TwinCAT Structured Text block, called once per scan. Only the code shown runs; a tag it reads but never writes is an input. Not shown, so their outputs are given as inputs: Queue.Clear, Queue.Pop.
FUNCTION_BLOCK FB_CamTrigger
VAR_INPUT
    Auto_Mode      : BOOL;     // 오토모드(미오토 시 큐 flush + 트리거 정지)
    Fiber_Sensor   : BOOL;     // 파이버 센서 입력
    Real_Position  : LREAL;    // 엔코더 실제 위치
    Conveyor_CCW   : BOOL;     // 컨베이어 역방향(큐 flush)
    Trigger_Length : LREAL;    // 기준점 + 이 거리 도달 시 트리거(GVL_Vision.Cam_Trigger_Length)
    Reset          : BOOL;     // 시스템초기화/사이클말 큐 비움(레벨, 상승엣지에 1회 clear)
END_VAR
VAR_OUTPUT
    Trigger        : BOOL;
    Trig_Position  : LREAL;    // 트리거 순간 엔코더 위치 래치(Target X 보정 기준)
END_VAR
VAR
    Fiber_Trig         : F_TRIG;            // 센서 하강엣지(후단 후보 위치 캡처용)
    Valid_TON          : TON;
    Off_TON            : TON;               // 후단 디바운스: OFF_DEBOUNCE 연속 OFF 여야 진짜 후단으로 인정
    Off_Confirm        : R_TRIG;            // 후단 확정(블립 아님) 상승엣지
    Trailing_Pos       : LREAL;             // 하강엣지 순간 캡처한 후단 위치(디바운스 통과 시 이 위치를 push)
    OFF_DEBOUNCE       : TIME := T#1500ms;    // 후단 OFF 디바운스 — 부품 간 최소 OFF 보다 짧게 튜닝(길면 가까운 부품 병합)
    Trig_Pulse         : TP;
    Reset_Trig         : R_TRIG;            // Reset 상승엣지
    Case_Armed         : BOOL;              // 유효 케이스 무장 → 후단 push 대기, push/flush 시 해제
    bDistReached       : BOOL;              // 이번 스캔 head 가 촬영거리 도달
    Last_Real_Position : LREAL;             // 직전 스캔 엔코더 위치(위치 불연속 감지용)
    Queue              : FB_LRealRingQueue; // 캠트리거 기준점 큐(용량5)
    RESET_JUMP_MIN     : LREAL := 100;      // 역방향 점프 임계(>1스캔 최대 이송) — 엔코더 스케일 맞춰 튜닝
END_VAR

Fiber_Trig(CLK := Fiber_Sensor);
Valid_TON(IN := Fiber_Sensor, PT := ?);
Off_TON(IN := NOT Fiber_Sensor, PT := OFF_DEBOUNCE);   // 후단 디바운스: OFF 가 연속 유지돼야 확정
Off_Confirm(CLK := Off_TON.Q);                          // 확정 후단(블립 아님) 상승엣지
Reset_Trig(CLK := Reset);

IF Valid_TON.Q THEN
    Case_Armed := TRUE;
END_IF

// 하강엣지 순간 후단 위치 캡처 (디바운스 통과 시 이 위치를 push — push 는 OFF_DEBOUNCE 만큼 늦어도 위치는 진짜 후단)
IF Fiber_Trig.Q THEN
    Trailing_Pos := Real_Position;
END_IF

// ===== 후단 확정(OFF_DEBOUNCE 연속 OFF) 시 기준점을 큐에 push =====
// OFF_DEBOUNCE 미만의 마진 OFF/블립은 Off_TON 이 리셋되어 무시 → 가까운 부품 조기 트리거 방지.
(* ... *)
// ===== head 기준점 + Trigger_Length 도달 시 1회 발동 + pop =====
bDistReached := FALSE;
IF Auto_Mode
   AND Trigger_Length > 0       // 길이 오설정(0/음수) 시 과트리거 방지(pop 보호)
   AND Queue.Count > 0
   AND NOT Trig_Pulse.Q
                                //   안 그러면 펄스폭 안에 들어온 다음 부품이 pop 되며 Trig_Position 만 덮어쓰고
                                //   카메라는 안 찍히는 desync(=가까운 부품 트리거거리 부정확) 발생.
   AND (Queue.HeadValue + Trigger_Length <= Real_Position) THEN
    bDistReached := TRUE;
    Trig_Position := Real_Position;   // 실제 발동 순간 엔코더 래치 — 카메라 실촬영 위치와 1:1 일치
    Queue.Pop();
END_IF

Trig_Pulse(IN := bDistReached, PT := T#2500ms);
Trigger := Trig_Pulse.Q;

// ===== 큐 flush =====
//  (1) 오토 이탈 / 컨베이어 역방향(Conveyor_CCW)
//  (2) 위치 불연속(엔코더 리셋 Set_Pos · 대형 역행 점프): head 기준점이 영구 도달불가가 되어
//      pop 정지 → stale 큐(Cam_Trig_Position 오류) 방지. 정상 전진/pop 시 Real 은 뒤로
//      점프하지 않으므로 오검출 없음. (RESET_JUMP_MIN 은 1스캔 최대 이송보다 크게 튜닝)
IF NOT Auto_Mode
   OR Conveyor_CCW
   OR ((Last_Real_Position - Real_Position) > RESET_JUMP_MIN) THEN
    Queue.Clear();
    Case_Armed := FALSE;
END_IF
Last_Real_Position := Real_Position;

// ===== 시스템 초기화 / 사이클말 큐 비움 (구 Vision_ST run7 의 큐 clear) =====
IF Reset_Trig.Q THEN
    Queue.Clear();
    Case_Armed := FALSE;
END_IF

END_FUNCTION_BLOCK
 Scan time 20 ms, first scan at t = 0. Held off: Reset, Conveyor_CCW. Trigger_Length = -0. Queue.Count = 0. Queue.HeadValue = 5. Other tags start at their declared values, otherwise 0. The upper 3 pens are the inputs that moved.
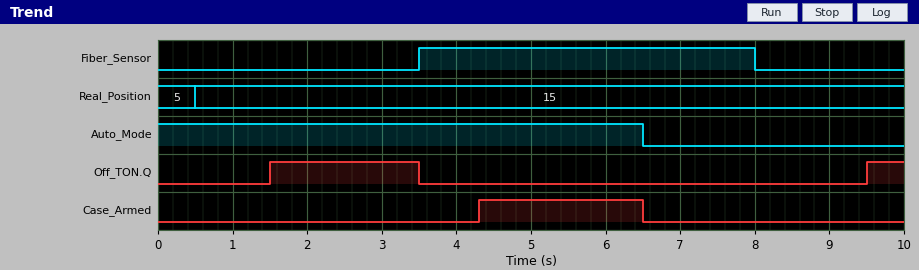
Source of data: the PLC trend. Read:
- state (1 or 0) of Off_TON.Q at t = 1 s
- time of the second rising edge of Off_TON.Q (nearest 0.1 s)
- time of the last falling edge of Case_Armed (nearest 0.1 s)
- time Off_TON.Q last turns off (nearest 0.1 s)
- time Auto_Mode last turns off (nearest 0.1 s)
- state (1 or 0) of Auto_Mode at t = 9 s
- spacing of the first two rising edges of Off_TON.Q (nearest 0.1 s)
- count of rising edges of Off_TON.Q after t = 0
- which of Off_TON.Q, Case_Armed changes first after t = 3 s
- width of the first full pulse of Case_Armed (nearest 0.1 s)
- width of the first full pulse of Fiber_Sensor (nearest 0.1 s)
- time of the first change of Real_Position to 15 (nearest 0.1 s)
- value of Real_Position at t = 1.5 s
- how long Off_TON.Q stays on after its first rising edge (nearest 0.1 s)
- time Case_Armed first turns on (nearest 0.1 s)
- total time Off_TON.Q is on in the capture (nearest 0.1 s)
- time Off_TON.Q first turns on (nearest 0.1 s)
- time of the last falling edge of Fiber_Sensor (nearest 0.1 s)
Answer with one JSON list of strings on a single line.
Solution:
["0", "9.5 s", "6.5 s", "3.5 s", "6.5 s", "0", "8.0 s", "2", "Off_TON.Q", "2.2 s", "4.5 s", "0.5 s", "15", "2.0 s", "4.3 s", "2.5 s", "1.5 s", "8.0 s"]
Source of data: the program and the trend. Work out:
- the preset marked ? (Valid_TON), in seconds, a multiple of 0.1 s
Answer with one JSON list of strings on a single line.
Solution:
["0.8 s"]
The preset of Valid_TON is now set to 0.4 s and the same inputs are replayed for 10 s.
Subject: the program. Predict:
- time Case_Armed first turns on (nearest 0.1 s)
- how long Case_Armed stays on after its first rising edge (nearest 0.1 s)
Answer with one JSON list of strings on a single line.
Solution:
["3.9 s", "2.6 s"]
